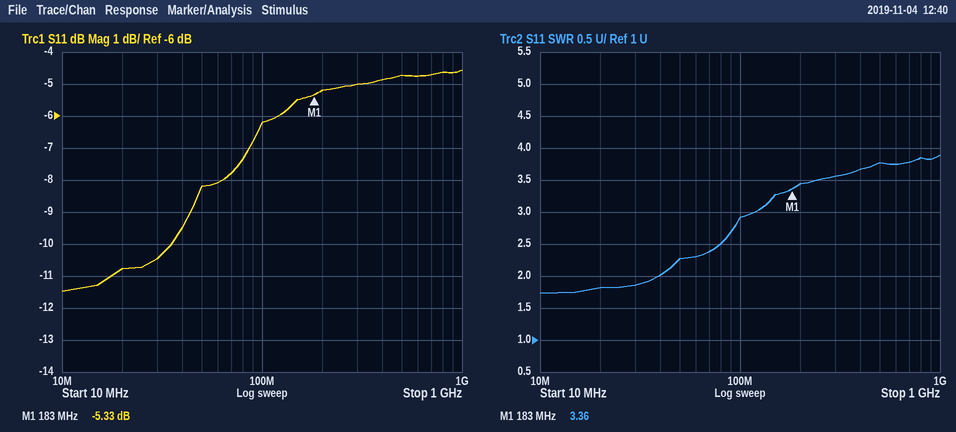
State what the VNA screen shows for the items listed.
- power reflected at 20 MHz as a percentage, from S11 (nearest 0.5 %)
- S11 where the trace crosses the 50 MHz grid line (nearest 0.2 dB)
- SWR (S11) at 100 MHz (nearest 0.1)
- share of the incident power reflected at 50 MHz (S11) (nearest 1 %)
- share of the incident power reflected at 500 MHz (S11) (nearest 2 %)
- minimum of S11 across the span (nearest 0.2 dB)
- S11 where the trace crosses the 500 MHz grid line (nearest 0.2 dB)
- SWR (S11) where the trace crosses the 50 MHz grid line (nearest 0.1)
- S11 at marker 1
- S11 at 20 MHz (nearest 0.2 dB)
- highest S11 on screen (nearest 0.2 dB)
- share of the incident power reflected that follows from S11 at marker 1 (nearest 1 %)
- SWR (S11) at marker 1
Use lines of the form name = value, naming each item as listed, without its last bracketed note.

power reflected at 20 MHz as a percentage, from S11 = 8.5 %
S11 where the trace crosses the 50 MHz grid line = -8.2 dB
SWR (S11) at 100 MHz = 2.9
share of the incident power reflected at 50 MHz (S11) = 15 %
share of the incident power reflected at 500 MHz (S11) = 34 %
minimum of S11 across the span = -11.4 dB
S11 where the trace crosses the 500 MHz grid line = -4.8 dB
SWR (S11) where the trace crosses the 50 MHz grid line = 2.3
S11 at marker 1 = -5.33 dB
S11 at 20 MHz = -10.8 dB
highest S11 on screen = -4.6 dB
share of the incident power reflected that follows from S11 at marker 1 = 29 %
SWR (S11) at marker 1 = 3.36
